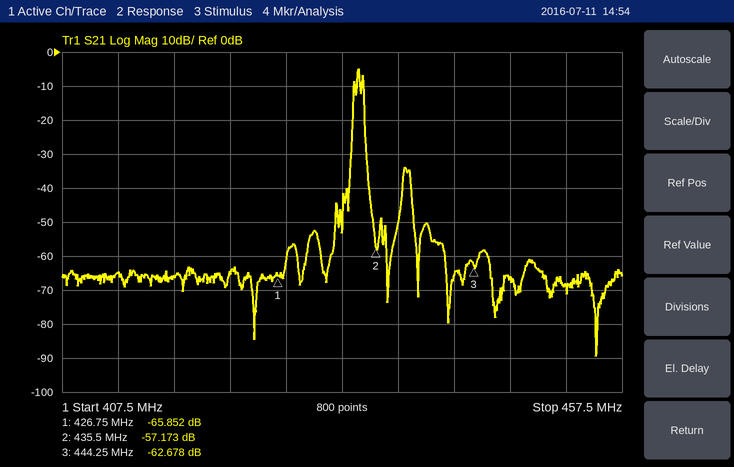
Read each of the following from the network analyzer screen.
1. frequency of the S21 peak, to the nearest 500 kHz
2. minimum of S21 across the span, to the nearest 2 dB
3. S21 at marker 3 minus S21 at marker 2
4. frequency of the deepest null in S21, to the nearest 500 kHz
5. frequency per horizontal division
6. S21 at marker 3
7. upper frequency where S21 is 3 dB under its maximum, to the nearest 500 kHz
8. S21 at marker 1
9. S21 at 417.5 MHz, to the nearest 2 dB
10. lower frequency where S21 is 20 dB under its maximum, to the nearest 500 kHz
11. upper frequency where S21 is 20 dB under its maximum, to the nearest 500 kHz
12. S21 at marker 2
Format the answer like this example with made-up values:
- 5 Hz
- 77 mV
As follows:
- 434.0 MHz
- -90 dB
- -5.505 dB
- 455.0 MHz
- 5 MHz
- -62.678 dB
- 434.0 MHz
- -65.852 dB
- -66 dB
- 433.5 MHz
- 434.5 MHz
- -57.173 dB
